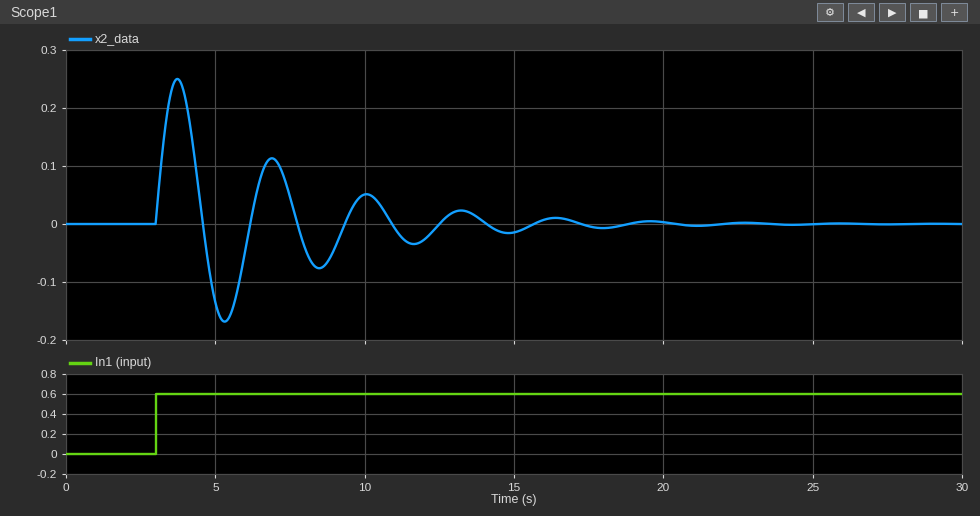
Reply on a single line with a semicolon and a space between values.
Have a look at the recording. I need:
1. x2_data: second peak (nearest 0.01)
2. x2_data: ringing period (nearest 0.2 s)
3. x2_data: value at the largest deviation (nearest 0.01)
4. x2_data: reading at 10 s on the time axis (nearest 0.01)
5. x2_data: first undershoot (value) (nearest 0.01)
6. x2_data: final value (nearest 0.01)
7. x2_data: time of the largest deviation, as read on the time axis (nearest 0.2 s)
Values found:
0.11; 3.2 s; 0.25; 0.05; -0.17; 0.00; 3.8 s
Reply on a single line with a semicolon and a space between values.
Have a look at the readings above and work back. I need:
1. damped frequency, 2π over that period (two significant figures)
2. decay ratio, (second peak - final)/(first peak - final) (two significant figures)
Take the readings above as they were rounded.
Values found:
2.0 rad/s; 0.44
